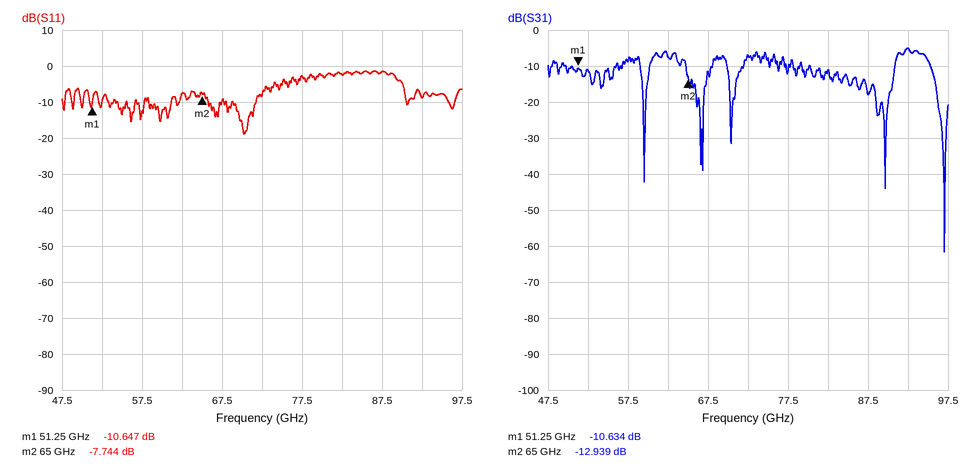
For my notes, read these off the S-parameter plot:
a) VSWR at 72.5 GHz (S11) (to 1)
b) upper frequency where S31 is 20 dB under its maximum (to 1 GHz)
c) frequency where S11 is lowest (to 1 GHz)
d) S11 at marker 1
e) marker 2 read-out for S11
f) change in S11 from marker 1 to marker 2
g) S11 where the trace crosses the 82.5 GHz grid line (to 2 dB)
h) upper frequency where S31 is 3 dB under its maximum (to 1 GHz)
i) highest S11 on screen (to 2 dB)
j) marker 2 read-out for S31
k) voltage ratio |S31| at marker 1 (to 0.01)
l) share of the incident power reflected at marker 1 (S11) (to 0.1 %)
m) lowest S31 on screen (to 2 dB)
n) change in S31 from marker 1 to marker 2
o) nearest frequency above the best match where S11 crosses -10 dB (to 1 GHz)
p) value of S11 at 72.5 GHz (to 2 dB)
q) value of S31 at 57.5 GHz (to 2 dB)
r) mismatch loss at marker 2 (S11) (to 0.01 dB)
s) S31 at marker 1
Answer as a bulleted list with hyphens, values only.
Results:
- 2
- 97 GHz
- 70 GHz
- -10.647 dB
- -7.744 dB
- 2.903 dB
- -2 dB
- 95 GHz
- -2 dB
- -12.939 dB
- 0.29
- 8.6 %
- -62 dB
- -2.305 dB
- 72 GHz
- -8 dB
- -8 dB
- 0.80 dB
- -10.634 dB
